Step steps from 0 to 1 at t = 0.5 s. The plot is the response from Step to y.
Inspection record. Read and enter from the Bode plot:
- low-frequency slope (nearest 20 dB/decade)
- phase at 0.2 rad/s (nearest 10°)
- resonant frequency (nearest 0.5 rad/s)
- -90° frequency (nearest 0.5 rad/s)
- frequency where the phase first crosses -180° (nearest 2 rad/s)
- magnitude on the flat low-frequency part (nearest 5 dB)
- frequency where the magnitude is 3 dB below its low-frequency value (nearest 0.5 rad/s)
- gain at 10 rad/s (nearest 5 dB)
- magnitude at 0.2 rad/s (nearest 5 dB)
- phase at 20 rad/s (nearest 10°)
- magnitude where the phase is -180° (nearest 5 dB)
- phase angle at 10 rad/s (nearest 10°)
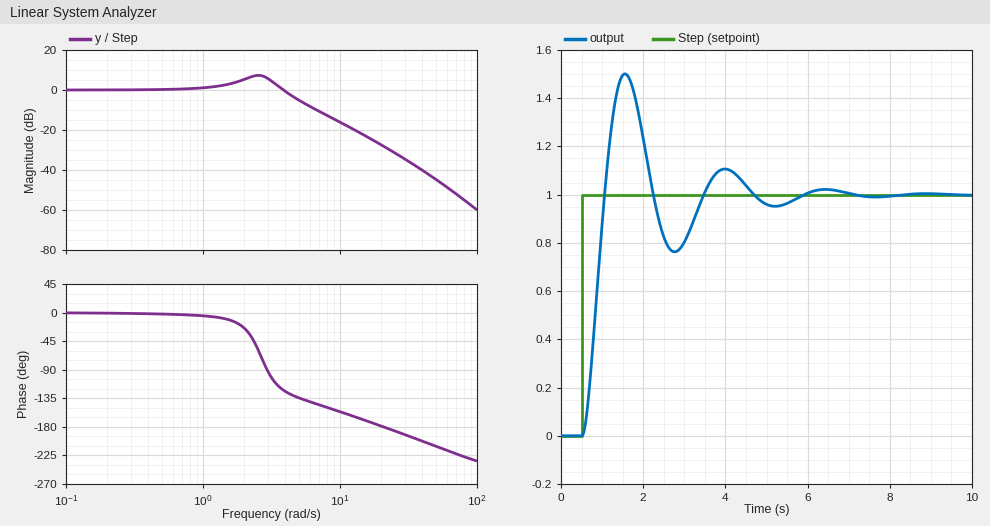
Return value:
0 dB/decade
0°
2.5 rad/s
3.0 rad/s
20 rad/s
0 dB
4.5 rad/s
-15 dB
0 dB
-180°
-30 dB
-160°
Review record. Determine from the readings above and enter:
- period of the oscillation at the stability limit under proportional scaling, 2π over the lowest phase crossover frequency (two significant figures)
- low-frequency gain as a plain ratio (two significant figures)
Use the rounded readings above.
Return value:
0.31 s
1.0
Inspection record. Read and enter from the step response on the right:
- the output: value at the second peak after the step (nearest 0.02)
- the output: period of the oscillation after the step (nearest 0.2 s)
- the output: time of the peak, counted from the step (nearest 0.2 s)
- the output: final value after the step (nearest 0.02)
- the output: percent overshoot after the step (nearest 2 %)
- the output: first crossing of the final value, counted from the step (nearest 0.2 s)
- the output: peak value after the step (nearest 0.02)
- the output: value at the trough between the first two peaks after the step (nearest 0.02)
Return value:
1.10
2.4 s
1.0 s
1.00
50 %
0.6 s
1.50
0.76
